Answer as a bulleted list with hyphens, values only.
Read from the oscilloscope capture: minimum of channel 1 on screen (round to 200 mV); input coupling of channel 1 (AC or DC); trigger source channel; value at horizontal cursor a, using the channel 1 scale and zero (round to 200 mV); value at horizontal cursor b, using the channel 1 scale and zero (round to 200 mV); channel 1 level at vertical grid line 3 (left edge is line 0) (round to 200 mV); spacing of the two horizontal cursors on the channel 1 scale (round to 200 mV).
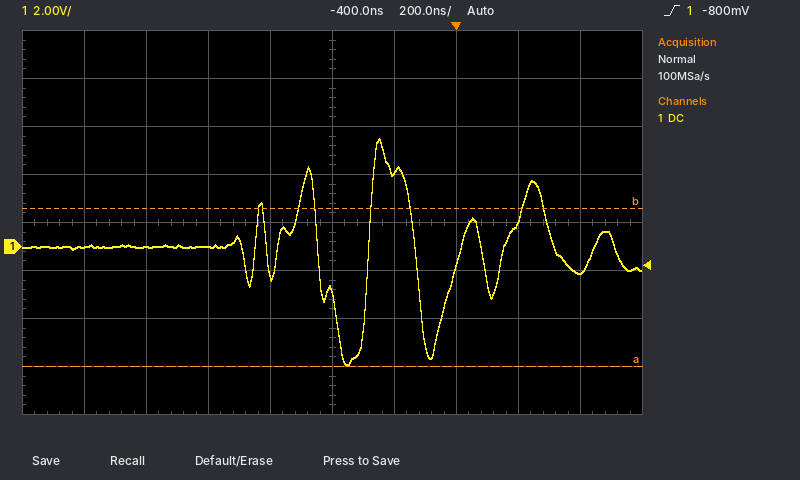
- -5.0 V
- DC
- channel 1
- -5.0 V
- 1.6 V
- 0.0 V
- 6.6 V
